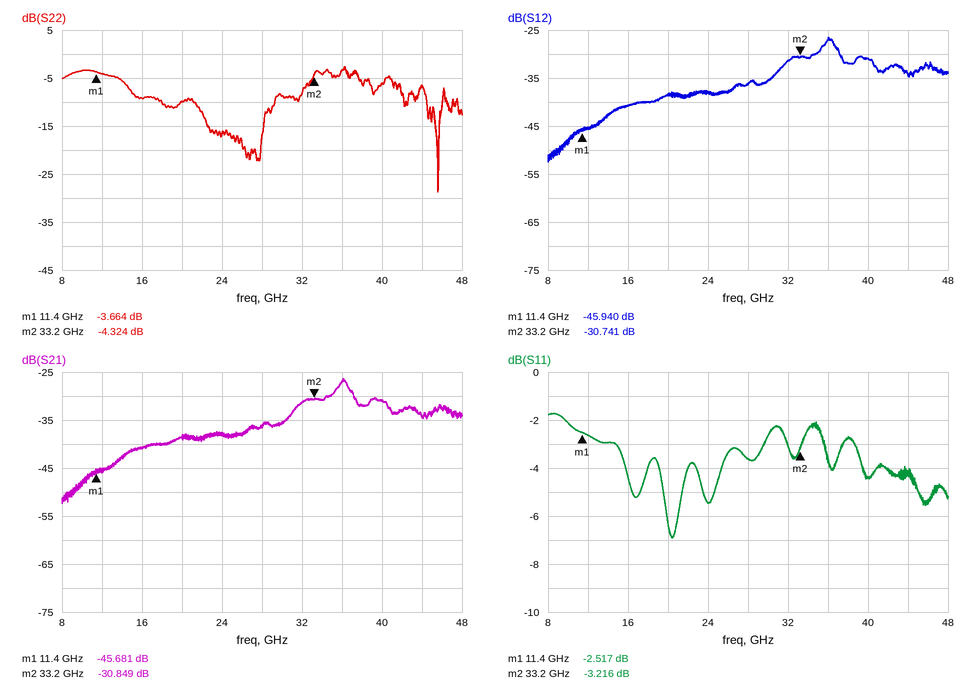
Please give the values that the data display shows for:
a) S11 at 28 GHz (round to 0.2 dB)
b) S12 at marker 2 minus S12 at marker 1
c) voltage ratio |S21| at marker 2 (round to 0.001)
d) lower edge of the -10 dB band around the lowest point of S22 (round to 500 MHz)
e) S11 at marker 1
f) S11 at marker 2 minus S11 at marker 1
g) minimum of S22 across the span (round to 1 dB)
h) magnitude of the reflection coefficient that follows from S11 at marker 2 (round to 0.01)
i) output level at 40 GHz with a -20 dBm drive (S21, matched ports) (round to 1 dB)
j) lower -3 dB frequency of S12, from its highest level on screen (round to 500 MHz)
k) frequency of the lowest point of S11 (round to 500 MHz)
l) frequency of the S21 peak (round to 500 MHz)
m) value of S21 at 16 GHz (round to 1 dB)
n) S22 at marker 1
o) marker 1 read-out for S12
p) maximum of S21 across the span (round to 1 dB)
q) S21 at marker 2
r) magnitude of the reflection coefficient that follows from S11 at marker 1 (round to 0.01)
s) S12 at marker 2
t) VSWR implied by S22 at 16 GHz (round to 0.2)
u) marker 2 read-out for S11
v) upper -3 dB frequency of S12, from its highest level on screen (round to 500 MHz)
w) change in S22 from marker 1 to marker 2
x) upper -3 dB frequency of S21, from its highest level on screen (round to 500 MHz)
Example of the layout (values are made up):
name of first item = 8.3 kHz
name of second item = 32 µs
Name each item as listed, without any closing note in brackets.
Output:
S11 at 28 GHz = -3.6 dB
S12 at marker 2 minus S12 at marker 1 = 15.199 dB
voltage ratio |S21| at marker 2 = 0.029
lower edge of the -10 dB band around the lowest point of S22 = 44.5 GHz
S11 at marker 1 = -2.517 dB
S11 at marker 2 minus S11 at marker 1 = -0.699 dB
minimum of S22 across the span = -29 dB
magnitude of the reflection coefficient that follows from S11 at marker 2 = 0.69
output level at 40 GHz with a -20 dBm drive (S21, matched ports) = -51 dBm
lower -3 dB frequency of S12, from its highest level on screen = 35.0 GHz
frequency of the lowest point of S11 = 20.5 GHz
frequency of the S21 peak = 36.0 GHz
value of S21 at 16 GHz = -41 dB
S22 at marker 1 = -3.664 dB
marker 1 read-out for S12 = -45.940 dB
maximum of S21 across the span = -26 dB
S21 at marker 2 = -30.849 dB
magnitude of the reflection coefficient that follows from S11 at marker 1 = 0.75
S12 at marker 2 = -30.741 dB
VSWR implied by S22 at 16 GHz = 2.0
marker 2 read-out for S11 = -3.216 dB
upper -3 dB frequency of S12, from its highest level on screen = 37.0 GHz
change in S22 from marker 1 to marker 2 = -0.660 dB
upper -3 dB frequency of S21, from its highest level on screen = 37.0 GHz
